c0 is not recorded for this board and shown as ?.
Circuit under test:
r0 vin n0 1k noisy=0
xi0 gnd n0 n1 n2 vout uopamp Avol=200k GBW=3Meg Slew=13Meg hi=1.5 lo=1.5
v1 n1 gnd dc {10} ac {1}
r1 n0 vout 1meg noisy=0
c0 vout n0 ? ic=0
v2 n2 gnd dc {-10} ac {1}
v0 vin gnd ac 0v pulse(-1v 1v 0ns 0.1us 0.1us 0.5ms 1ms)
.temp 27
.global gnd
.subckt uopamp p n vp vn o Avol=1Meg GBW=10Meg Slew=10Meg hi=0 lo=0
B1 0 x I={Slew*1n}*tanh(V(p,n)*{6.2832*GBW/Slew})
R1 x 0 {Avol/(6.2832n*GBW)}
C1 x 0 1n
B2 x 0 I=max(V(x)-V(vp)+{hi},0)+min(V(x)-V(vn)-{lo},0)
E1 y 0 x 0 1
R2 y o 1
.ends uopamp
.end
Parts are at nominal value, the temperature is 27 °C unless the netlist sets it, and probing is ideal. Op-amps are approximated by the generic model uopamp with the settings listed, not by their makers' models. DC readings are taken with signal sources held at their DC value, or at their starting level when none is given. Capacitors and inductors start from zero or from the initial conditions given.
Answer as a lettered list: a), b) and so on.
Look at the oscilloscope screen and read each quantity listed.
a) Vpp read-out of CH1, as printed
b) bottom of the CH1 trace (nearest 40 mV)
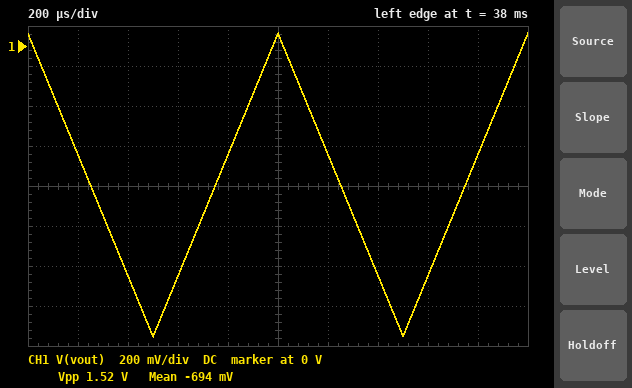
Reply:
a) 1.52 V
b) -1.44 V
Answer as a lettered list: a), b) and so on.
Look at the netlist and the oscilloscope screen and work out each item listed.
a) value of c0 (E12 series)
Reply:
a) 330 nF
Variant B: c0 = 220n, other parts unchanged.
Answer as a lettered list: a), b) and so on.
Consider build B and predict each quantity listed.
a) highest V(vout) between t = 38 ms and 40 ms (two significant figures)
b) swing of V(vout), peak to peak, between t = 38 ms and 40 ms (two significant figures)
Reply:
a) 160 mV
b) 2.3 V
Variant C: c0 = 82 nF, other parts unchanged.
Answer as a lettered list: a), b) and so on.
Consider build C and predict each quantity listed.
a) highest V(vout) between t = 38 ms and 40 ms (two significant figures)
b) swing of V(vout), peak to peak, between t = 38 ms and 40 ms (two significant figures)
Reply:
a) 1.1 V
b) 6.1 V
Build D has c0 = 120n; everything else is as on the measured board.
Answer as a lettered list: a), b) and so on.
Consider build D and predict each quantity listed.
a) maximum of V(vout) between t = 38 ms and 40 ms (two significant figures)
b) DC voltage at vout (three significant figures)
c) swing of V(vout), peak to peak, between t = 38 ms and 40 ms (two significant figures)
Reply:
a) 540 mV
b) 8.51 V
c) 4.2 V
